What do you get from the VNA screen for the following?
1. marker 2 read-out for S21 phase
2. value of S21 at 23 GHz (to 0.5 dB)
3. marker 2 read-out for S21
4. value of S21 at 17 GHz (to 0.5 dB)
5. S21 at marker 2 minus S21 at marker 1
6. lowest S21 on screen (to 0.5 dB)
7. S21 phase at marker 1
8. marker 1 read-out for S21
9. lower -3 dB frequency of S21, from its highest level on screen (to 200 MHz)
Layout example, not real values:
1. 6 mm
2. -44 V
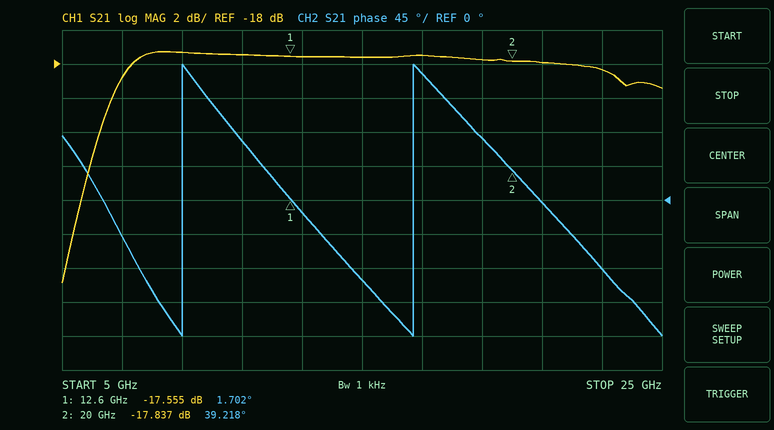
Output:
1. 39.218°
2. -18.5 dB
3. -17.837 dB
4. -17.5 dB
5. -0.282 dB
6. -31.0 dB
7. 1.702°
8. -17.555 dB
9. 6.6 GHz
